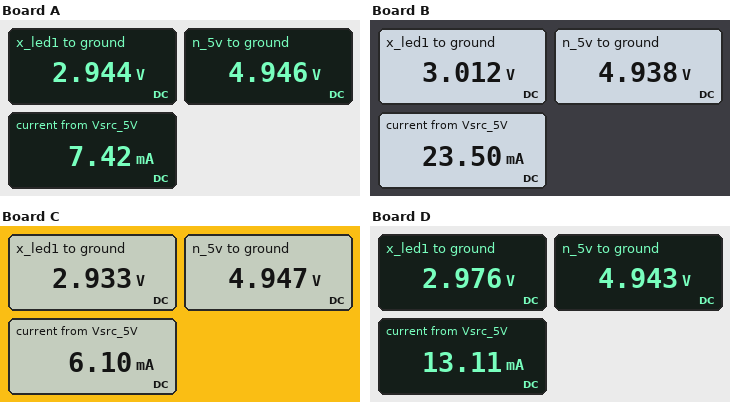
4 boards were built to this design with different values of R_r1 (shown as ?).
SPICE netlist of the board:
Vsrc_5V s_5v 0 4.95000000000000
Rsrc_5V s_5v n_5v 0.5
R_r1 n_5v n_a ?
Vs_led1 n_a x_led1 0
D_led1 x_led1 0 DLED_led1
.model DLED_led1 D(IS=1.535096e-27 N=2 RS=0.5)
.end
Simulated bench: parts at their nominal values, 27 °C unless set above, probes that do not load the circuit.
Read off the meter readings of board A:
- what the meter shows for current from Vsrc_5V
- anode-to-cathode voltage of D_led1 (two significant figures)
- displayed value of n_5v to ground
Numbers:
7.42 mA
2.9 V
4.946 V
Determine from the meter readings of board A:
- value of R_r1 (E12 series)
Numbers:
270 Ω
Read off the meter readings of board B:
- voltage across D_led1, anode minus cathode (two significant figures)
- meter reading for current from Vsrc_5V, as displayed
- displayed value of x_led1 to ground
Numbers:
3.0 V
23.50 mA
3.012 V
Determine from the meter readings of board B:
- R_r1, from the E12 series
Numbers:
82 Ω
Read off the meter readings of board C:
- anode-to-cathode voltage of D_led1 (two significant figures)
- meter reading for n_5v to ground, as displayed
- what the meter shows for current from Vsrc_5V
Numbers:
2.9 V
4.947 V
6.10 mA
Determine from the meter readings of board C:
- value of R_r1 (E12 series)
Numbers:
330 Ω
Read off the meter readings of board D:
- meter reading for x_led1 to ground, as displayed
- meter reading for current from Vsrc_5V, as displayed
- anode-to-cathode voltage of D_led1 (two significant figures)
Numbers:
2.976 V
13.11 mA
3.0 V
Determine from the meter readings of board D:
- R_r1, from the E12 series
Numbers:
150 Ω
